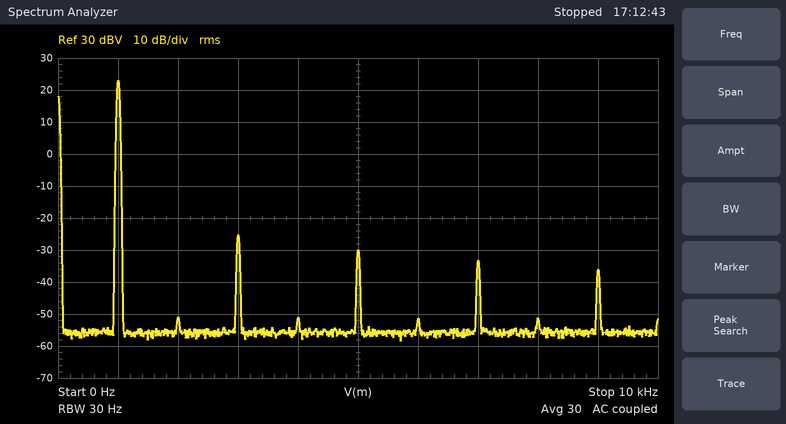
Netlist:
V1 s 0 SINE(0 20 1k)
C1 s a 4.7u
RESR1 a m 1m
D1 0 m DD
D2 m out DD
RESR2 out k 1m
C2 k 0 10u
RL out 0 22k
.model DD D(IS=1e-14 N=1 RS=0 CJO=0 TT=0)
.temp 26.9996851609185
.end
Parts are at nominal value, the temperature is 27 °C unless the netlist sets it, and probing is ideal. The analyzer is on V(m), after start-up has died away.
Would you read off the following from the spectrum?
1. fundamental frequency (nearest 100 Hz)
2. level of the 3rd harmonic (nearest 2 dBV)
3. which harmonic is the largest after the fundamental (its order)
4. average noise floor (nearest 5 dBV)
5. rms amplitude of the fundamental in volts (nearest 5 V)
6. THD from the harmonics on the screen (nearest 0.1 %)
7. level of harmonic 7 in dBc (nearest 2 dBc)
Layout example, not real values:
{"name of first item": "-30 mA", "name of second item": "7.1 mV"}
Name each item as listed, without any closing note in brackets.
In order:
{"fundamental frequency": "1.0 kHz", "level of the 3rd harmonic": "-26 dBV", "which harmonic is the largest after the fundamental": "3", "average noise floor": "-55 dBV", "rms amplitude of the fundamental in volts": "15 V", "THD from the harmonics on the screen": "0.5 %", "level of harmonic 7 in dBc": "-56 dBc"}
